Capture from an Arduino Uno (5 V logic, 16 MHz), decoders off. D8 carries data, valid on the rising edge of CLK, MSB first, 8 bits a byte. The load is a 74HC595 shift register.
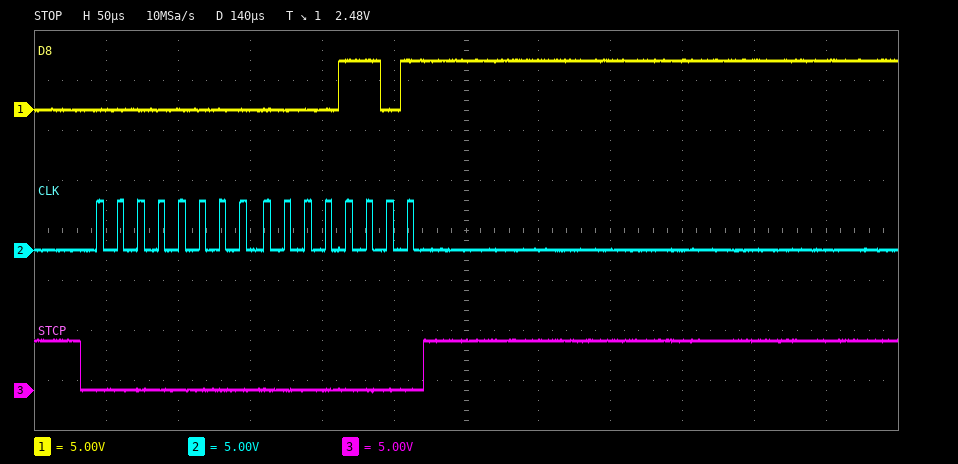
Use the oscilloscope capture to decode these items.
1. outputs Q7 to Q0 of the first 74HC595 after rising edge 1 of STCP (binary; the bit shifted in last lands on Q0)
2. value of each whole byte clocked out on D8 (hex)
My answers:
00001101
00 0D
